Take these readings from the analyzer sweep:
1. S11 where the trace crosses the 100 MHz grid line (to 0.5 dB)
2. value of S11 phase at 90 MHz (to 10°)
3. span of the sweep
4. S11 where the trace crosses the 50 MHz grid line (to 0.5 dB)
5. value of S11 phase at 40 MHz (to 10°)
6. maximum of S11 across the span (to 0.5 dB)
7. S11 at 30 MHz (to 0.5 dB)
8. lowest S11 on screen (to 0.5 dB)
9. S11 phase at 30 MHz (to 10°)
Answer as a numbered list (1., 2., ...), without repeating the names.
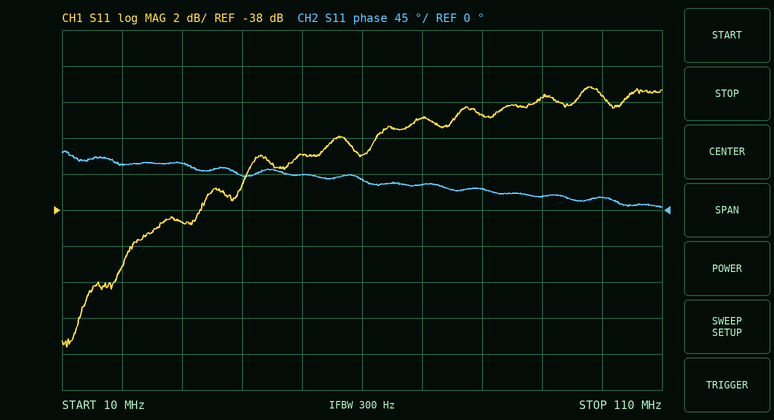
1. -31.5 dB
2. 20°
3. 100 MHz
4. -35.0 dB
5. 40°
6. -31.0 dB
7. -38.5 dB
8. -45.5 dB
9. 60°
